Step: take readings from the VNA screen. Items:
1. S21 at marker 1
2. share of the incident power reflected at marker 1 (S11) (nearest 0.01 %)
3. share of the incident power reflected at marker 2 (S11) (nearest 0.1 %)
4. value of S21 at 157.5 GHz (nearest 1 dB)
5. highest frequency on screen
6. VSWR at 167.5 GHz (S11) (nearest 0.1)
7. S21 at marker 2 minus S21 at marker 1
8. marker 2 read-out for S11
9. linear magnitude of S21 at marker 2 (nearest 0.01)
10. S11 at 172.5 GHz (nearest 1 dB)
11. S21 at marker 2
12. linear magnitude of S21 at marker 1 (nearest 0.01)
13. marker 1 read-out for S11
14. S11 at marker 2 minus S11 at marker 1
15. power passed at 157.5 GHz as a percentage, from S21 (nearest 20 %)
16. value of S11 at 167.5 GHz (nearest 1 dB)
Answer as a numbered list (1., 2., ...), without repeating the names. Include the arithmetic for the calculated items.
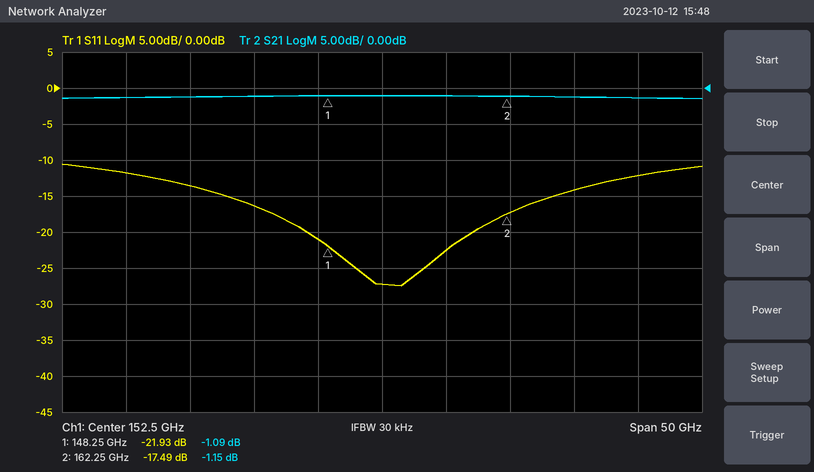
1. -1.09 dB
2. 10^(-21.93/10) ≈ 0.64 %
3. 10^(-17.49/10) ≈ 1.8 %
4. -1 dB
5. 177.5 GHz
6. |Γ| = 10^(-14/20) = 0.1995; VSWR = (1 + 0.1995)/(1 − 0.1995) ≈ 1.5
7. -1.15 − (-1.09) = -0.06 dB
8. -17.49 dB
9. 10^(-1.15/20) ≈ 0.88
10. -12 dB
11. -1.15 dB
12. 10^(-1.09/20) ≈ 0.88
13. -21.93 dB
14. -17.49 − (-21.93) = 4.44 dB
15. 10^(-1/10) ≈ 79.4 %, so 80 % to the nearest 20 %
16. -14 dB
